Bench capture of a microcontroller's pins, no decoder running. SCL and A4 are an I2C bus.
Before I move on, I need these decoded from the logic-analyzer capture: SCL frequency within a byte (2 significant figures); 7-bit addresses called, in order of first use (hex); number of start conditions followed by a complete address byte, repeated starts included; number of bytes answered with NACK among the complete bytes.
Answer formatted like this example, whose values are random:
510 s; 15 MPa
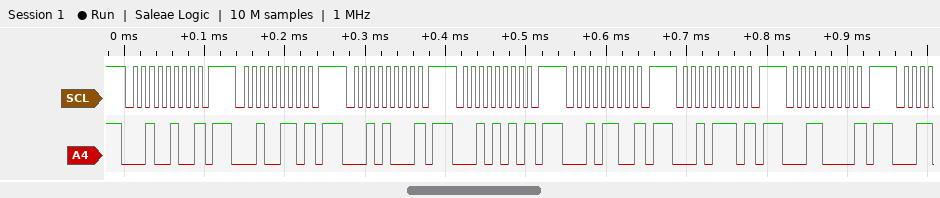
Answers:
100 kHz; 0x12 0x13 0x14 0x15 0x16 0x17 0x18; 7; 7
